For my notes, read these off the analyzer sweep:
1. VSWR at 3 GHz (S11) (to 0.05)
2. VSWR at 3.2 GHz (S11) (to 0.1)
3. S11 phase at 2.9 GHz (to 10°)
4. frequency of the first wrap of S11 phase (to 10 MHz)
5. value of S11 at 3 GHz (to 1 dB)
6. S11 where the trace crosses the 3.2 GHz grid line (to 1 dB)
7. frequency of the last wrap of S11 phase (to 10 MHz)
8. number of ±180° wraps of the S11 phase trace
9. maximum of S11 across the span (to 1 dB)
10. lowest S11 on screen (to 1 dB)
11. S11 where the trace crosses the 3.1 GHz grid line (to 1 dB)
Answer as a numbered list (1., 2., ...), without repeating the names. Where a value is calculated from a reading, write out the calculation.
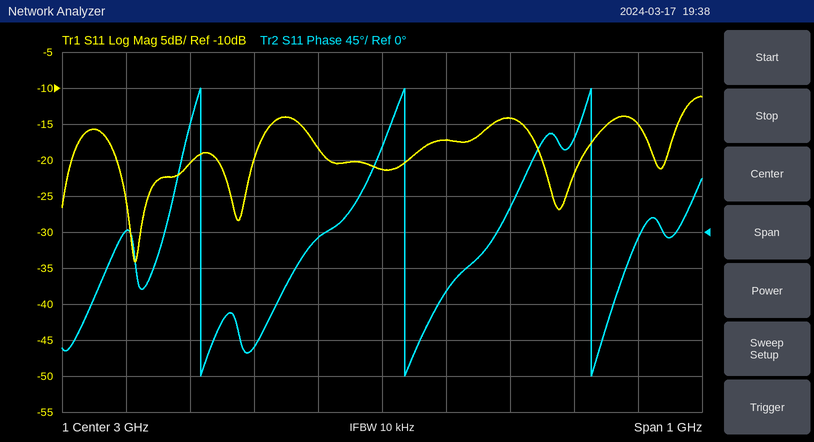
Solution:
1. |Γ| = 10^(-21/20) = 0.0891; VSWR = (1 + 0.0891)/(1 − 0.0891) ≈ 1.20
2. |Γ| = 10^(-14/20) = 0.1995; VSWR = (1 + 0.1995)/(1 − 0.1995) ≈ 1.5
3. -10°
4. 2.72 GHz
5. -21 dB
6. -14 dB
7. 3.33 GHz
8. 3
9. -11 dB
10. -34 dB
11. -17 dB
